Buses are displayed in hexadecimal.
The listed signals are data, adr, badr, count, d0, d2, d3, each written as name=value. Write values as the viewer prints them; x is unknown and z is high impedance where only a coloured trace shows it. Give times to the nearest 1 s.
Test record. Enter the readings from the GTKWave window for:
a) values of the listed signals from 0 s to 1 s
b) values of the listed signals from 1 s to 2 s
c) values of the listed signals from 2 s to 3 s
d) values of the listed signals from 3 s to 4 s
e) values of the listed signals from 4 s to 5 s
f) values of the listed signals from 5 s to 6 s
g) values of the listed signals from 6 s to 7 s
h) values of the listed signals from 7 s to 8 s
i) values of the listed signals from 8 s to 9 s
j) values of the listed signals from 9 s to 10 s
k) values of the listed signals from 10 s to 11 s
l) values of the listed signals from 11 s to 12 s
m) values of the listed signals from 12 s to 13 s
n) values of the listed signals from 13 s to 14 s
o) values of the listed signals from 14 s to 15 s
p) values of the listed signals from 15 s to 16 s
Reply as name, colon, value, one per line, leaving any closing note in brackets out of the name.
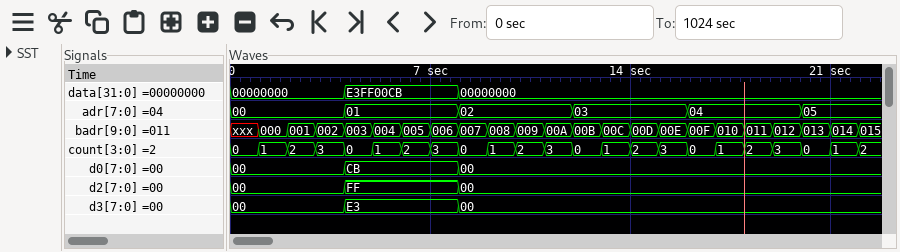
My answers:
values of the listed signals from 0 s to 1 s: data=00000000, adr=00, badr=xxx, count=0, d0=00, d2=00, d3=00
values of the listed signals from 1 s to 2 s: data=00000000, adr=00, badr=000, count=1, d0=00, d2=00, d3=00
values of the listed signals from 2 s to 3 s: data=00000000, adr=00, badr=001, count=2, d0=00, d2=00, d3=00
values of the listed signals from 3 s to 4 s: data=00000000, adr=00, badr=002, count=3, d0=00, d2=00, d3=00
values of the listed signals from 4 s to 5 s: data=E3FF00CB, adr=01, badr=003, count=0, d0=CB, d2=FF, d3=E3
values of the listed signals from 5 s to 6 s: data=E3FF00CB, adr=01, badr=004, count=1, d0=CB, d2=FF, d3=E3
values of the listed signals from 6 s to 7 s: data=E3FF00CB, adr=01, badr=005, count=2, d0=CB, d2=FF, d3=E3
values of the listed signals from 7 s to 8 s: data=E3FF00CB, adr=01, badr=006, count=3, d0=CB, d2=FF, d3=E3
values of the listed signals from 8 s to 9 s: data=00000000, adr=02, badr=007, count=0, d0=00, d2=00, d3=00
values of the listed signals from 9 s to 10 s: data=00000000, adr=02, badr=008, count=1, d0=00, d2=00, d3=00
values of the listed signals from 10 s to 11 s: data=00000000, adr=02, badr=009, count=2, d0=00, d2=00, d3=00
values of the listed signals from 11 s to 12 s: data=00000000, adr=02, badr=00A, count=3, d0=00, d2=00, d3=00
values of the listed signals from 12 s to 13 s: data=00000000, adr=03, badr=00B, count=0, d0=00, d2=00, d3=00
values of the listed signals from 13 s to 14 s: data=00000000, adr=03, badr=00C, count=1, d0=00, d2=00, d3=00
values of the listed signals from 14 s to 15 s: data=00000000, adr=03, badr=00D, count=2, d0=00, d2=00, d3=00
values of the listed signals from 15 s to 16 s: data=00000000, adr=03, badr=00E, count=3, d0=00, d2=00, d3=00
